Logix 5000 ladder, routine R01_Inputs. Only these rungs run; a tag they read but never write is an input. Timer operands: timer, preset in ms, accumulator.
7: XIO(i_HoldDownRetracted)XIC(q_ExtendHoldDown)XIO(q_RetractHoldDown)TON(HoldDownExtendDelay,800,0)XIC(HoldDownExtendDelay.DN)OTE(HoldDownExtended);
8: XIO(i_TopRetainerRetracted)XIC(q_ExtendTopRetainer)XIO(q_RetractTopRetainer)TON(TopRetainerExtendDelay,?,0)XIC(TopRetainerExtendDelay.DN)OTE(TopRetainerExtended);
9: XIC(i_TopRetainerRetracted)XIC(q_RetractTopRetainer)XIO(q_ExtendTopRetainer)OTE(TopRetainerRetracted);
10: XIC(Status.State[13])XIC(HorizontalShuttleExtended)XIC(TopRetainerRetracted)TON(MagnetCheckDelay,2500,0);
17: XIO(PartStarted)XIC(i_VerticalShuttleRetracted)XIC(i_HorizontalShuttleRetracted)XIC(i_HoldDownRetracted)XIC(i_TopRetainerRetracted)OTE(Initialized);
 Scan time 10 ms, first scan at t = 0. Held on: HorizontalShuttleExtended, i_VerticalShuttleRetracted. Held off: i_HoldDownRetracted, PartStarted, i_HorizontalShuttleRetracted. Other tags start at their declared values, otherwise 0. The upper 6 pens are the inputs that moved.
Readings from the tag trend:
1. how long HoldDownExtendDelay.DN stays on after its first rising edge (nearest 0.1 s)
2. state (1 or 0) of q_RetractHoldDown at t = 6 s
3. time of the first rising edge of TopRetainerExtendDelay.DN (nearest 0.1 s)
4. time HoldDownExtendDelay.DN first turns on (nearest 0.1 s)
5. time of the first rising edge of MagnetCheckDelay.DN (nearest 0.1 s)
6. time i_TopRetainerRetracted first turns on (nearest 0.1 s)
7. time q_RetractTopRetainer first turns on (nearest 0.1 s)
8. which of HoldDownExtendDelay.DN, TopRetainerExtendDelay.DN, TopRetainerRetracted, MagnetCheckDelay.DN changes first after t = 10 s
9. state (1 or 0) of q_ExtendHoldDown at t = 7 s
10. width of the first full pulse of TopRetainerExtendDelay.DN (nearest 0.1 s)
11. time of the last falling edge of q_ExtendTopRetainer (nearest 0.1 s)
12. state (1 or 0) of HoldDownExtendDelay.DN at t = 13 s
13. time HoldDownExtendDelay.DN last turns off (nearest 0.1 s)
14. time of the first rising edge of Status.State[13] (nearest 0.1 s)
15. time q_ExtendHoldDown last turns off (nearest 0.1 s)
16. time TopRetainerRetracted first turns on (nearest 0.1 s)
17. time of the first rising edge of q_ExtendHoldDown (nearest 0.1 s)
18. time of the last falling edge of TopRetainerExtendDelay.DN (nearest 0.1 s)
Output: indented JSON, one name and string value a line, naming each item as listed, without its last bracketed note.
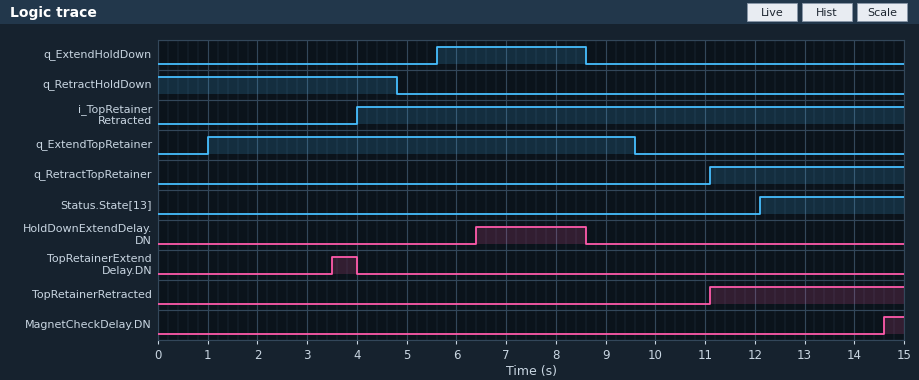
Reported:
{
  "how long HoldDownExtendDelay.DN stays on after its first rising edge": "2.2 s",
  "state (1 or 0) of q_RetractHoldDown at t = 6 s": "0",
  "time of the first rising edge of TopRetainerExtendDelay.DN": "3.5 s",
  "time HoldDownExtendDelay.DN first turns on": "6.4 s",
  "time of the first rising edge of MagnetCheckDelay.DN": "14.6 s",
  "time i_TopRetainerRetracted first turns on": "4.0 s",
  "time q_RetractTopRetainer first turns on": "11.1 s",
  "which of HoldDownExtendDelay.DN, TopRetainerExtendDelay.DN, TopRetainerRetracted, MagnetCheckDelay.DN changes first after t = 10 s": "TopRetainerRetracted",
  "state (1 or 0) of q_ExtendHoldDown at t = 7 s": "1",
  "width of the first full pulse of TopRetainerExtendDelay.DN": "0.5 s",
  "time of the last falling edge of q_ExtendTopRetainer": "9.6 s",
  "state (1 or 0) of HoldDownExtendDelay.DN at t = 13 s": "0",
  "time HoldDownExtendDelay.DN last turns off": "8.6 s",
  "time of the first rising edge of Status.State[13]": "12.1 s",
  "time q_ExtendHoldDown last turns off": "8.6 s",
  "time TopRetainerRetracted first turns on": "11.1 s",
  "time of the first rising edge of q_ExtendHoldDown": "5.6 s",
  "time of the last falling edge of TopRetainerExtendDelay.DN": "4.0 s"
}
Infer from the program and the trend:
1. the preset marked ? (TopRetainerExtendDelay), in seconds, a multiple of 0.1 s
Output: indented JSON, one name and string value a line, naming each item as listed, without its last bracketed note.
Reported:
{
  "the preset marked ? (TopRetainerExtendDelay), in seconds, a multiple of 0.1 s": "2.5 s"
}
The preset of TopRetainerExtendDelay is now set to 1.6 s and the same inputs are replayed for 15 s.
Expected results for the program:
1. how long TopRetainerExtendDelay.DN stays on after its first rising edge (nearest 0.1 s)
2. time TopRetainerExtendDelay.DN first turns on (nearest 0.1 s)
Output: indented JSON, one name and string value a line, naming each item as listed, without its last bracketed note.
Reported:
{
  "how long TopRetainerExtendDelay.DN stays on after its first rising edge": "1.4 s",
  "time TopRetainerExtendDelay.DN first turns on": "2.6 s"
}
